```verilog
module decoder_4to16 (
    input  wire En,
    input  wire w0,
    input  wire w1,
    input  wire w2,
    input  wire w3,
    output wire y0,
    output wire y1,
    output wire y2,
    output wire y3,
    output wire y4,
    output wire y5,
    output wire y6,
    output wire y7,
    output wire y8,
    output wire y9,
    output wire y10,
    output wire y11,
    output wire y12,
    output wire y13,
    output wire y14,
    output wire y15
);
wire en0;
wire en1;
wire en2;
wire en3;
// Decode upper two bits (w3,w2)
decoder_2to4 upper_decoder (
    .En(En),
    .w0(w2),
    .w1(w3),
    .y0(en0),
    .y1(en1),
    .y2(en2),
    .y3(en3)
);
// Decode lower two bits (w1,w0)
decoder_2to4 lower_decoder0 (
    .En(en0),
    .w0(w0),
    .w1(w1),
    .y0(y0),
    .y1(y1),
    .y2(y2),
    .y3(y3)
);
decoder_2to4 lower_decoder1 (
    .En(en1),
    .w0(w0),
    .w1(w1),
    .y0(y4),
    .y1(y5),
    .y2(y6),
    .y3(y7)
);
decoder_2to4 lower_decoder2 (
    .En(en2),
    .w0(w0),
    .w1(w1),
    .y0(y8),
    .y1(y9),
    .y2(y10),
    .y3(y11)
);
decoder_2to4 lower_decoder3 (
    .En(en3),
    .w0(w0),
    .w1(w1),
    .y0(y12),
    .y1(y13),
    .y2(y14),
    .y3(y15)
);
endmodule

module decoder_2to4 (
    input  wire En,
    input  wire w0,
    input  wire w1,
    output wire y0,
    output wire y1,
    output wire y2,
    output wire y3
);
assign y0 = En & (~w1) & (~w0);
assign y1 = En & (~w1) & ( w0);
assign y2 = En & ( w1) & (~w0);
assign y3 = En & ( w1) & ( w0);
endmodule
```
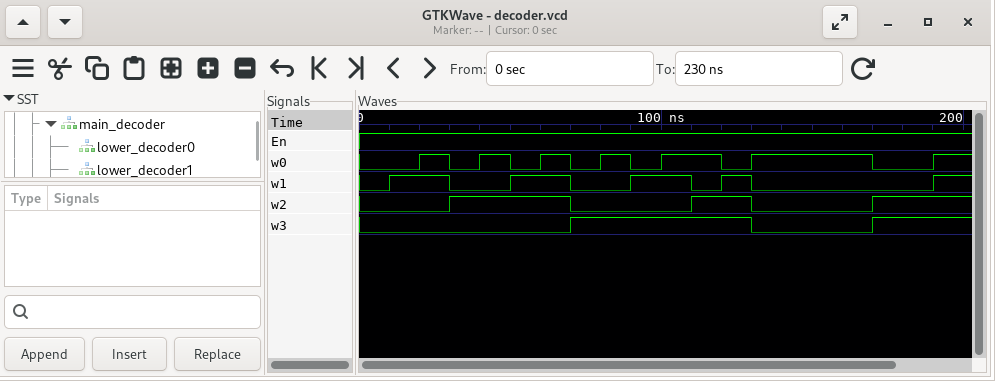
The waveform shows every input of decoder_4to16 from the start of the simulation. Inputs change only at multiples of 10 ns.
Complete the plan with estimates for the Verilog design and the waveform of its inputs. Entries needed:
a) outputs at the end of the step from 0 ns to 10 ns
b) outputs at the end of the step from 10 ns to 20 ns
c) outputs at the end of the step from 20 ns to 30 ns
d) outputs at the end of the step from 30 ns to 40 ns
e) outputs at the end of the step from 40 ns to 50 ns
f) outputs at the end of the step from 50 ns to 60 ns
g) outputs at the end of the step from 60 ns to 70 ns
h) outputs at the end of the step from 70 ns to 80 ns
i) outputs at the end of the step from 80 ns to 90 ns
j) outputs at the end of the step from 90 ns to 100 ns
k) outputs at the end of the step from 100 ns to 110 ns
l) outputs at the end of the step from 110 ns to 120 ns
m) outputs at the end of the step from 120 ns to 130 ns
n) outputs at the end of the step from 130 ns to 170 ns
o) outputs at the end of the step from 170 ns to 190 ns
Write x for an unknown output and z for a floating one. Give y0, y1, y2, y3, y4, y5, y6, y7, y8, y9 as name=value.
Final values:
y0=1, y1=0, y2=0, y3=0, y4=0, y5=0, y6=0, y7=0, y8=0, y9=0
y0=0, y1=0, y2=1, y3=0, y4=0, y5=0, y6=0, y7=0, y8=0, y9=0
y0=0, y1=0, y2=0, y3=1, y4=0, y5=0, y6=0, y7=0, y8=0, y9=0
y0=0, y1=0, y2=0, y3=0, y4=1, y5=0, y6=0, y7=0, y8=0, y9=0
y0=0, y1=0, y2=0, y3=0, y4=0, y5=1, y6=0, y7=0, y8=0, y9=0
y0=0, y1=0, y2=0, y3=0, y4=0, y5=0, y6=1, y7=0, y8=0, y9=0
y0=0, y1=0, y2=0, y3=0, y4=0, y5=0, y6=0, y7=1, y8=0, y9=0
y0=0, y1=0, y2=0, y3=0, y4=0, y5=0, y6=0, y7=0, y8=1, y9=0
y0=0, y1=0, y2=0, y3=0, y4=0, y5=0, y6=0, y7=0, y8=0, y9=1
y0=0, y1=0, y2=0, y3=0, y4=0, y5=0, y6=0, y7=0, y8=0, y9=0
y0=0, y1=0, y2=0, y3=0, y4=0, y5=0, y6=0, y7=0, y8=0, y9=0
y0=0, y1=0, y2=0, y3=0, y4=0, y5=0, y6=0, y7=0, y8=0, y9=0
y0=0, y1=0, y2=0, y3=0, y4=0, y5=0, y6=0, y7=0, y8=0, y9=0
y0=0, y1=1, y2=0, y3=0, y4=0, y5=0, y6=0, y7=0, y8=0, y9=0
y0=0, y1=0, y2=0, y3=0, y4=0, y5=0, y6=0, y7=0, y8=0, y9=0
